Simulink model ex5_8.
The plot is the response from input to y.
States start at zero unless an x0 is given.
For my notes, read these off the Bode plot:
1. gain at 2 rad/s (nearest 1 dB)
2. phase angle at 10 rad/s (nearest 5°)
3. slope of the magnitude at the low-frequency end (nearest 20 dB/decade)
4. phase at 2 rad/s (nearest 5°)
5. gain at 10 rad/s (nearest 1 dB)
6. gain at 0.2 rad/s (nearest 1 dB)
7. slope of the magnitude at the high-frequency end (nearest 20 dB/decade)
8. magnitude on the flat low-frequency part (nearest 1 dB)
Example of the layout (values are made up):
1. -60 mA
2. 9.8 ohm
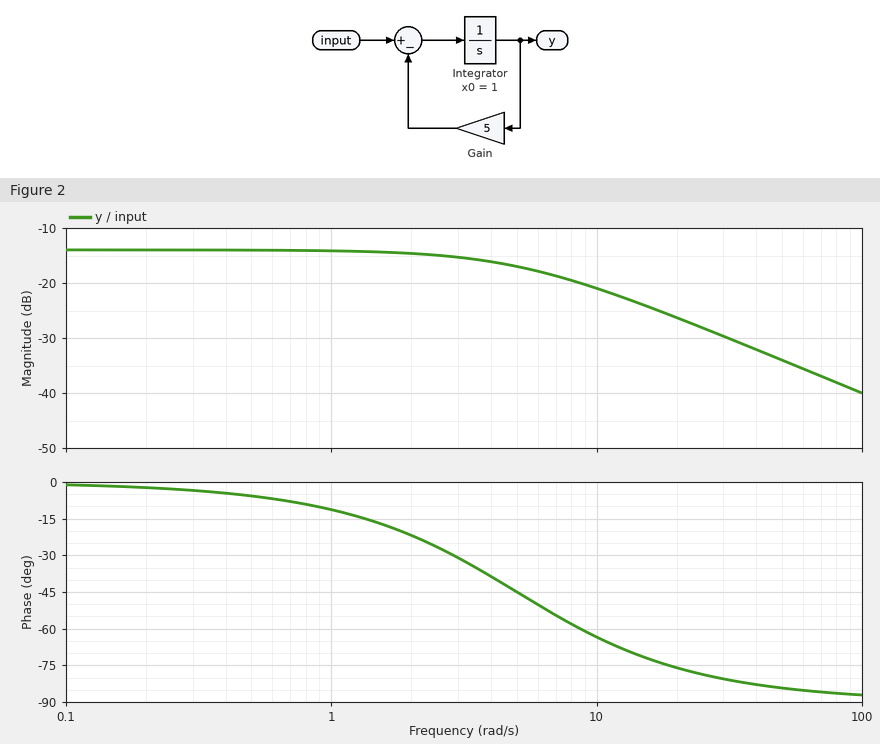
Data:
1. -15 dB
2. -65°
3. 0 dB/decade
4. -20°
5. -21 dB
6. -14 dB
7. -20 dB/decade
8. -14 dB
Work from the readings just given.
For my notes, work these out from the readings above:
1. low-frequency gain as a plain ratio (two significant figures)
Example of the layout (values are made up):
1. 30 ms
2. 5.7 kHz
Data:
1. 0.20
